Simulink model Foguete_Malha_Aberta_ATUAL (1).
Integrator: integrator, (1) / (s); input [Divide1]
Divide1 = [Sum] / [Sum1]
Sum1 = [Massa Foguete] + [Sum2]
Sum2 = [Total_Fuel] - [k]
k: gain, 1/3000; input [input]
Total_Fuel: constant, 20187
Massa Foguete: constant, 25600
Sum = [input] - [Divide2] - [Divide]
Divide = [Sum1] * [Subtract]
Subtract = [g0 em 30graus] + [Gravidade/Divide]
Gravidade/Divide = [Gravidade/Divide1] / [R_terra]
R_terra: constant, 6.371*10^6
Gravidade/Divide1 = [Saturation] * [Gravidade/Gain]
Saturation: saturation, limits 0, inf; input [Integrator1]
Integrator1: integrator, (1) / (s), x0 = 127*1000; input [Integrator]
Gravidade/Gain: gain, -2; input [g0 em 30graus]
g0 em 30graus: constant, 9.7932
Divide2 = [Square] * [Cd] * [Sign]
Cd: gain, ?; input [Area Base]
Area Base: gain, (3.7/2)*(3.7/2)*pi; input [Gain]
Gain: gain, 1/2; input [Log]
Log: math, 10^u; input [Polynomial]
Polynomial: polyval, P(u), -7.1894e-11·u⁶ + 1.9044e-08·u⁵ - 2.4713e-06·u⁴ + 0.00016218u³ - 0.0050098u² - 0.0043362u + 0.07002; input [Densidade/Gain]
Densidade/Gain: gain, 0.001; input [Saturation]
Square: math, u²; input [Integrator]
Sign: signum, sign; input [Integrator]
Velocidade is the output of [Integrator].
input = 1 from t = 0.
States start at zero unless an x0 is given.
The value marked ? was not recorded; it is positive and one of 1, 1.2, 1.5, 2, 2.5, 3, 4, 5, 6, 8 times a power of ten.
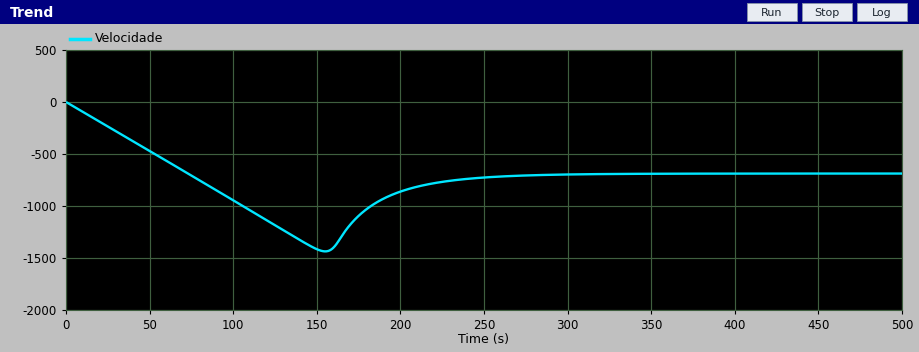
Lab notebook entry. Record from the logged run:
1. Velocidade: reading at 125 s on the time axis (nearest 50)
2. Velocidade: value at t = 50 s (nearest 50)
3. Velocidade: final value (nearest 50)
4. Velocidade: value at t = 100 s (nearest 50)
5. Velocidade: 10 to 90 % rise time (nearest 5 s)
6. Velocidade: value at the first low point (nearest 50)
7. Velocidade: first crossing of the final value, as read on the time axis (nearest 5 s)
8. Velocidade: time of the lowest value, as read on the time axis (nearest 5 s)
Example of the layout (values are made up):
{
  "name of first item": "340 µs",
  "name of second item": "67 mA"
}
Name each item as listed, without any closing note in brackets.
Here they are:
{
  "Velocidade: reading at 125 s on the time axis": "-1200",
  "Velocidade: value at t = 50 s": "-450",
  "Velocidade: final value": "-700",
  "Velocidade: value at t = 100 s": "-950",
  "Velocidade: 10 to 90 % rise time": "60 s",
  "Velocidade: value at the first low point": "-1450",
  "Velocidade: first crossing of the final value, as read on the time axis": "75 s",
  "Velocidade: time of the lowest value, as read on the time axis": "155 s"
}
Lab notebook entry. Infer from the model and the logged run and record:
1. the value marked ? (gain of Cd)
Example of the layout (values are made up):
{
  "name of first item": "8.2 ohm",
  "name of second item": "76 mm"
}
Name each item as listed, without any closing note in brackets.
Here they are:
{
  "the value marked ?": "0.15"
}
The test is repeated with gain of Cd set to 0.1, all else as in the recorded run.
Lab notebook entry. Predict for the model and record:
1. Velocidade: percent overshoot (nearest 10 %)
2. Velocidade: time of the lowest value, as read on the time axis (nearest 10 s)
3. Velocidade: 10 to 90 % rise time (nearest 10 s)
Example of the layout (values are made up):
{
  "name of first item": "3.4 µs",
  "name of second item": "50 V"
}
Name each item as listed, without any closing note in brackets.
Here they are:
{
  "Velocidade: percent overshoot": "70 %",
  "Velocidade: time of the lowest value, as read on the time axis": "160 s",
  "Velocidade: 10 to 90 % rise time": "70 s"
}
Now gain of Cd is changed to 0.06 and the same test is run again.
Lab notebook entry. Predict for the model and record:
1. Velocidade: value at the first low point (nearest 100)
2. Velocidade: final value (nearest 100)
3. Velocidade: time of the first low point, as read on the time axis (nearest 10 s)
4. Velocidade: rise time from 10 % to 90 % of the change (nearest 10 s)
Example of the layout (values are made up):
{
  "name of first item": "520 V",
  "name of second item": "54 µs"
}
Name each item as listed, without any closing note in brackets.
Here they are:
{
  "Velocidade: value at the first low point": "-1500",
  "Velocidade: final value": "-1100",
  "Velocidade: time of the first low point, as read on the time axis": "160 s",
  "Velocidade: rise time from 10 % to 90 % of the change": "90 s"
}
